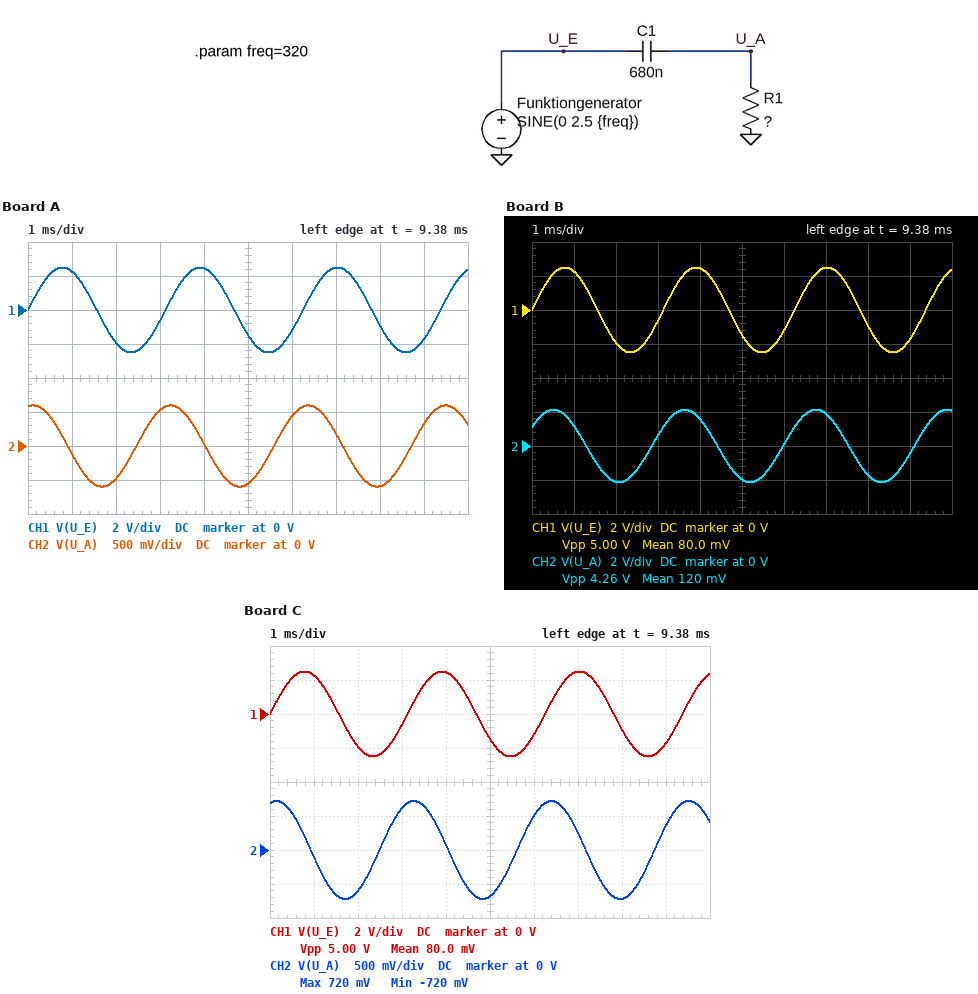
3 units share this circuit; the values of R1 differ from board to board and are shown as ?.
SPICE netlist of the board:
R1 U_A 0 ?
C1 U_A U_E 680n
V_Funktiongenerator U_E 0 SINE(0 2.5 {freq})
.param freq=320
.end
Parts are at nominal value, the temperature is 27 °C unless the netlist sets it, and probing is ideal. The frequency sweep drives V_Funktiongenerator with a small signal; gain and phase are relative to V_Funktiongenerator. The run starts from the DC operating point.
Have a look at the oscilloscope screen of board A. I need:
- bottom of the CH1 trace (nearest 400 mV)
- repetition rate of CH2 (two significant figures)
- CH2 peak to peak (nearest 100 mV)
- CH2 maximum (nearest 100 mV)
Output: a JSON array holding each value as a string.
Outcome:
["-2.4 V", "320 Hz", "1.2 V", "600 mV"]
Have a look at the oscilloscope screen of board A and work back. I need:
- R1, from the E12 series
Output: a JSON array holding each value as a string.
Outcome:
["180 Ω"]
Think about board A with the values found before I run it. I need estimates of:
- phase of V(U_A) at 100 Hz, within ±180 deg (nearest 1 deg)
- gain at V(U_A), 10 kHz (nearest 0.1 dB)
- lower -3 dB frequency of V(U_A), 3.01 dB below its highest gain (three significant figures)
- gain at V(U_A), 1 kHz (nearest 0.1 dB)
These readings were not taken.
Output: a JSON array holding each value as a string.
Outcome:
["86 deg", "-0.1 dB", "1.30 kHz", "-4.3 dB"]
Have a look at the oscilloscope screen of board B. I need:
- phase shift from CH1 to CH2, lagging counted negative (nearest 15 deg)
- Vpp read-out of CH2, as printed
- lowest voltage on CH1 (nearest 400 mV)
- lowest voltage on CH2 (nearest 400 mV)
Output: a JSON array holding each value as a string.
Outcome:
["30 deg", "4.26 V", "-2.4 V", "-2.0 V"]
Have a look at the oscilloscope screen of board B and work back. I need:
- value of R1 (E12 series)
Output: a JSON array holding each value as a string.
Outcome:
["1.2 kΩ"]
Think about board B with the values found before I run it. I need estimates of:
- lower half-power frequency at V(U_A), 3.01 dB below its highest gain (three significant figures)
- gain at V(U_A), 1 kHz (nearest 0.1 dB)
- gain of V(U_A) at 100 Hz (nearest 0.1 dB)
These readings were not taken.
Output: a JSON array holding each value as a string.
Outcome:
["195 Hz", "-0.2 dB", "-6.8 dB"]
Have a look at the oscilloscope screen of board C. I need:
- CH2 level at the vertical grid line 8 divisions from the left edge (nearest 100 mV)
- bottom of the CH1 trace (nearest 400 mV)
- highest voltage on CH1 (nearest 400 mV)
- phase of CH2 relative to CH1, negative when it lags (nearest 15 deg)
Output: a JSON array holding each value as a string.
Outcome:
["-700 mV", "-2.4 V", "2.4 V", "75 deg"]
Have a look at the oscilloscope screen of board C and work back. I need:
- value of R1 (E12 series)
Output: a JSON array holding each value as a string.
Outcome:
["220 Ω"]
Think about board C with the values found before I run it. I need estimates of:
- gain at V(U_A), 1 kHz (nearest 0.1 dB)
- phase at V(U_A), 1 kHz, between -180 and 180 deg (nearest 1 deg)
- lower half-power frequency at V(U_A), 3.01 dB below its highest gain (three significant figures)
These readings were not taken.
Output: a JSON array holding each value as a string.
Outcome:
["-3.3 dB", "47 deg", "1.06 kHz"]
